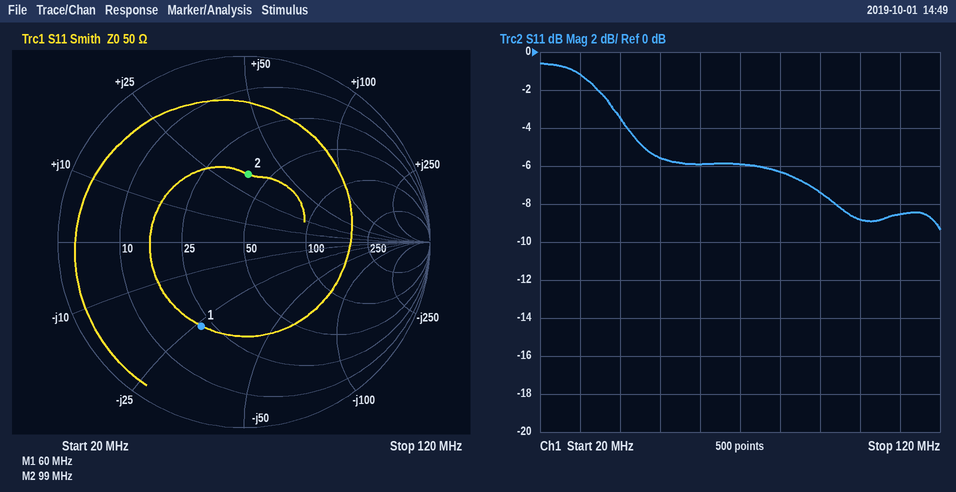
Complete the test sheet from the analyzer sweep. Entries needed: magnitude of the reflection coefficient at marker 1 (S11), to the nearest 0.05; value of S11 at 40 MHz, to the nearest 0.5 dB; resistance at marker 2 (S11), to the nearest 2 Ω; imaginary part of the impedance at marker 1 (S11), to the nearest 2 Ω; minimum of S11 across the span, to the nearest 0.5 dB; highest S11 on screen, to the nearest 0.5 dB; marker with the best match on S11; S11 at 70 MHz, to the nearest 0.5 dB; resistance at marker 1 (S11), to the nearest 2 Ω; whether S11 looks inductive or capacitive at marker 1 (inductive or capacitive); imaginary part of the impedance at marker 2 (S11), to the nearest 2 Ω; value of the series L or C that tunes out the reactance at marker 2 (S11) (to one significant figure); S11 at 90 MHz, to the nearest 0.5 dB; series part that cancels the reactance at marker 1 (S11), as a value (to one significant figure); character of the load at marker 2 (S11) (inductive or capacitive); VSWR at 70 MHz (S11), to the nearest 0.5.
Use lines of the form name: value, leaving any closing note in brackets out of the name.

magnitude of the reflection coefficient at marker 1 (S11), to the nearest 0.05: 0.50
value of S11 at 40 MHz, to the nearest 0.5 dB: -3.5 dB
resistance at marker 2 (S11), to the nearest 2 Ω: 40 Ω
imaginary part of the impedance at marker 1 (S11), to the nearest 2 Ω: -26 Ω
minimum of S11 across the span, to the nearest 0.5 dB: -9.5 dB
highest S11 on screen, to the nearest 0.5 dB: -0.5 dB
marker with the best match on S11: marker 2
S11 at 70 MHz, to the nearest 0.5 dB: -6.0 dB
resistance at marker 1 (S11), to the nearest 2 Ω: 22 Ω
whether S11 looks inductive or capacitive at marker 1: capacitive
imaginary part of the impedance at marker 2 (S11), to the nearest 2 Ω: +34 Ω
value of the series L or C that tunes out the reactance at marker 2 (S11): 50 pF
S11 at 90 MHz, to the nearest 0.5 dB: -7.5 dB
series part that cancels the reactance at marker 1 (S11), as a value: 70 nH
character of the load at marker 2 (S11): inductive
VSWR at 70 MHz (S11), to the nearest 0.5: 3.0
